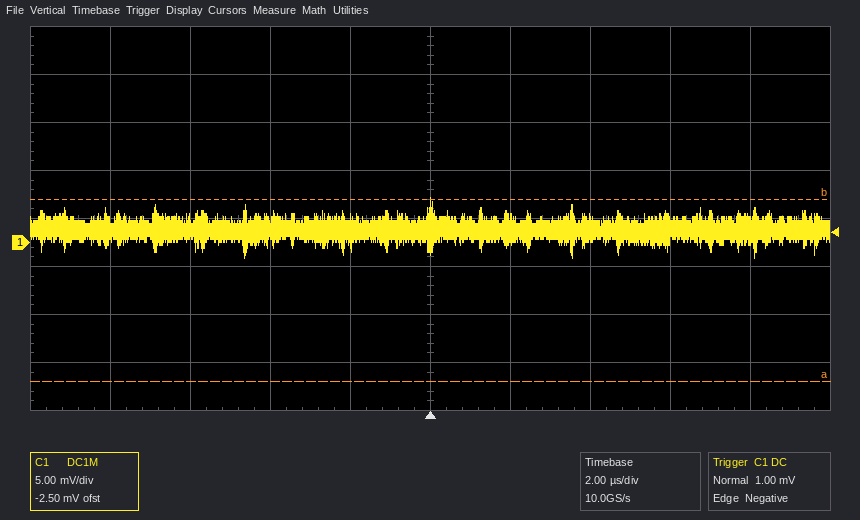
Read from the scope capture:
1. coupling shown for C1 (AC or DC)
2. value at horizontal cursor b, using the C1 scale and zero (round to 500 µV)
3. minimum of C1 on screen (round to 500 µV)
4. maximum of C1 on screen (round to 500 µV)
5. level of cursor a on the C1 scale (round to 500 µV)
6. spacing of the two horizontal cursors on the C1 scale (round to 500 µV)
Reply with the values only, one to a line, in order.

DC
4.5 mV
-1.5 mV
4.5 mV
-14.5 mV
19.0 mV
